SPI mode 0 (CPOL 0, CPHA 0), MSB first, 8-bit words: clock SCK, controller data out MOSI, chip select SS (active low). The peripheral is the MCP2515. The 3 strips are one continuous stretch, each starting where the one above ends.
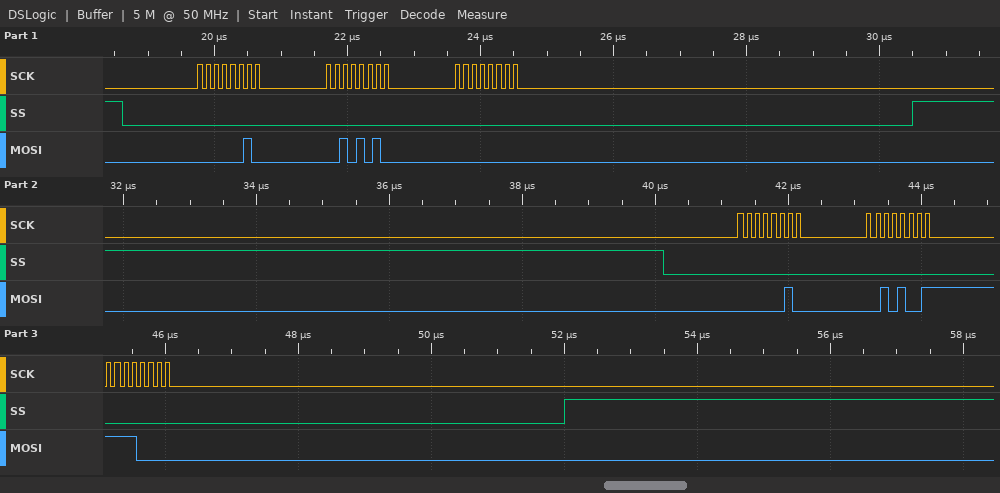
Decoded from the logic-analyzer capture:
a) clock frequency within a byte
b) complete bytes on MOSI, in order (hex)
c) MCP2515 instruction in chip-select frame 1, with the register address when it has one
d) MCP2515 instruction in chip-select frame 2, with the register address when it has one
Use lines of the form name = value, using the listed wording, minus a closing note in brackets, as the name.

clock frequency within a byte = 8 MHz
complete bytes on MOSI, in order = 0x02 0x2A 0x00 0x02 0x29 0xF0
MCP2515 instruction in chip-select frame 1, with the register address when it has one = WRITE 0x2A
MCP2515 instruction in chip-select frame 2, with the register address when it has one = WRITE 0x29
